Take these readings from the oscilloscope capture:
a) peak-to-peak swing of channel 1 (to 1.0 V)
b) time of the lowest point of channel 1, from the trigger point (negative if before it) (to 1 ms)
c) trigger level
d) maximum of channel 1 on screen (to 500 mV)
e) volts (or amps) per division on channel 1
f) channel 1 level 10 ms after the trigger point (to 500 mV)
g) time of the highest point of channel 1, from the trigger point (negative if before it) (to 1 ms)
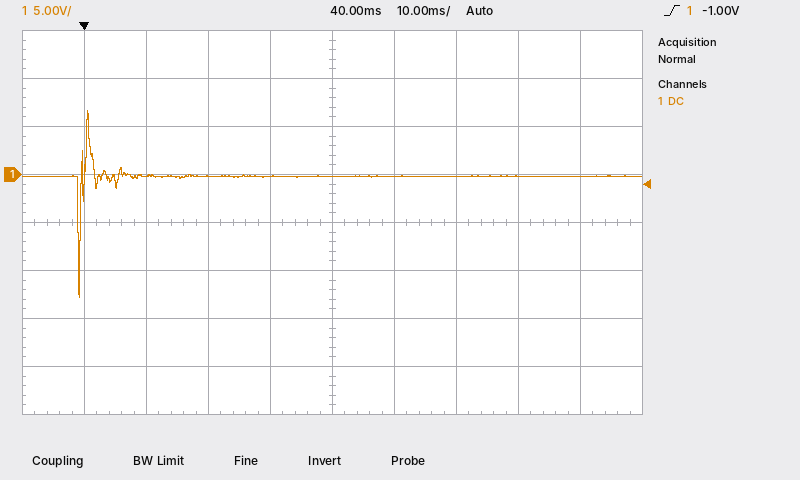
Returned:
19.0 V
-1 ms
-1.00 V
6.5 V
5 V
0.0 V
+1 ms
